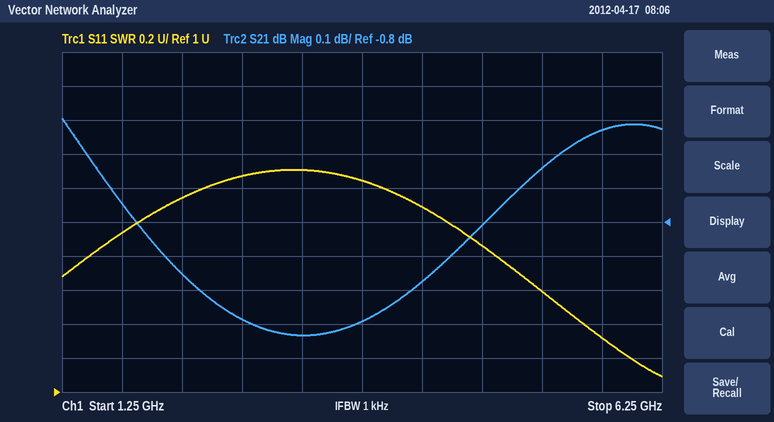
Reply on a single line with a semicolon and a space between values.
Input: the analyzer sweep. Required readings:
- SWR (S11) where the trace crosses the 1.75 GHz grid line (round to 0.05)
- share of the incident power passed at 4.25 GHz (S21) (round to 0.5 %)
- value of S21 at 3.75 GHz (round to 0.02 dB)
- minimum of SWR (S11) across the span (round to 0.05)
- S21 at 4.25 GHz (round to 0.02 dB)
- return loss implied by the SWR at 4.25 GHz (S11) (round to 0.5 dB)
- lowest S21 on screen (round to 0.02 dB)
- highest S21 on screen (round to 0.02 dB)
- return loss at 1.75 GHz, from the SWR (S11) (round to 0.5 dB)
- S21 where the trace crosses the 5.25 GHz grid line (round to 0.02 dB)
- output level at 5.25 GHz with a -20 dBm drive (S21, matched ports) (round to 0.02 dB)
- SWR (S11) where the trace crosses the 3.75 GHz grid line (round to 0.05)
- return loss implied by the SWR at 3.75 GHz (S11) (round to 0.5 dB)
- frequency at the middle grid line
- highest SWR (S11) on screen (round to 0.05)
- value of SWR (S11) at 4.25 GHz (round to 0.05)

1.95; 80.0 %; -1.10 dB; 1.10; -0.98 dB; 9.0 dB; -1.14 dB; -0.50 dB; 10.0 dB; -0.64 dB; -20.64 dBm; 2.25; 8.5 dB; 3.75 GHz; 2.30; 2.10
